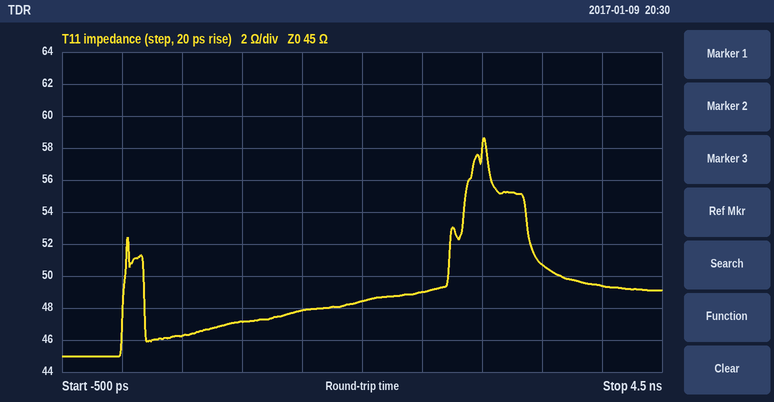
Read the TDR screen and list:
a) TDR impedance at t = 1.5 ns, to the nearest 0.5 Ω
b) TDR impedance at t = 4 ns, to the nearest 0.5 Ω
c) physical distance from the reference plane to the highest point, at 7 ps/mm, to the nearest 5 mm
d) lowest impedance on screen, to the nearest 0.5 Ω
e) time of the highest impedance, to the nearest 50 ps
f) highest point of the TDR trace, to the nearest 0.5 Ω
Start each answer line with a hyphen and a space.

- 48.0 Ω
- 49.5 Ω
- 215 mm
- 45.0 Ω
- 3.00 ns
- 58.5 Ω
